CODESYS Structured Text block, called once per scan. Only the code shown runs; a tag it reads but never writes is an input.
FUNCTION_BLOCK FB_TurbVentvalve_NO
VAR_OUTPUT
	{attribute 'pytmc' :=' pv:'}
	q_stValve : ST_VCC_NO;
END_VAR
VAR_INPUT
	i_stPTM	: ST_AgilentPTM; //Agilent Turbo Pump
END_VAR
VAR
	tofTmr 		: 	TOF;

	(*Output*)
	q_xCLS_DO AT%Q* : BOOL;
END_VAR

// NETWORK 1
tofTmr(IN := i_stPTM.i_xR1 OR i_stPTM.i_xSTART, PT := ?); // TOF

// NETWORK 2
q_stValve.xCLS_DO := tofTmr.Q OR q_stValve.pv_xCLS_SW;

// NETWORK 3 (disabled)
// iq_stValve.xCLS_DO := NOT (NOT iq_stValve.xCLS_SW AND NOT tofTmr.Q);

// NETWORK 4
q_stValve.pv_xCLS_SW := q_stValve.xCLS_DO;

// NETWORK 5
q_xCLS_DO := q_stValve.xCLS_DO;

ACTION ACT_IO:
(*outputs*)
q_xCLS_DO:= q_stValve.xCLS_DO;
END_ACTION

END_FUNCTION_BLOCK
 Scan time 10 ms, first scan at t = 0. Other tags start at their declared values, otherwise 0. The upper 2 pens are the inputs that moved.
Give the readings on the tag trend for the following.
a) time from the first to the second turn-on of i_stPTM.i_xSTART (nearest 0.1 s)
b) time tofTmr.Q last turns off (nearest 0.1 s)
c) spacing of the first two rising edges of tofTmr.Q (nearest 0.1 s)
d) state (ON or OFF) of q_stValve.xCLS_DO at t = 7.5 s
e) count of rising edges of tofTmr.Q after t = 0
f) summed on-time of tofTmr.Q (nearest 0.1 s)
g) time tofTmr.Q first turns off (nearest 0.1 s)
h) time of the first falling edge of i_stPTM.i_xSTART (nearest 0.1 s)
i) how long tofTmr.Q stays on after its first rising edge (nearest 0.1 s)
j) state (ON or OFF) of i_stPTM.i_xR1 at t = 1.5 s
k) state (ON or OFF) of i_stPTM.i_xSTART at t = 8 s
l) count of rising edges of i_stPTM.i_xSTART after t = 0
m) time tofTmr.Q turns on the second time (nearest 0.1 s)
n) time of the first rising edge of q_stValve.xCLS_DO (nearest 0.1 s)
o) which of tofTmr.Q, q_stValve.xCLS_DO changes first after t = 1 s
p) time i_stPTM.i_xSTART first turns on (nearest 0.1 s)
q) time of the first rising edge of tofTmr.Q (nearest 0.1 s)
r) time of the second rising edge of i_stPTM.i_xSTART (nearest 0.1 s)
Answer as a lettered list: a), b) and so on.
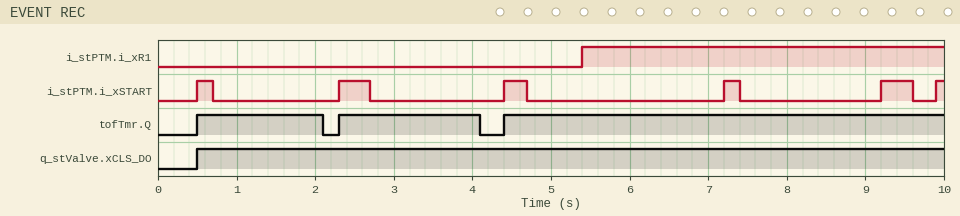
a) 1.8 s
b) 4.1 s
c) 1.8 s
d) ON
e) 3
f) 9.0 s
g) 2.1 s
h) 0.7 s
i) 1.6 s
j) OFF
k) OFF
l) 6
m) 2.3 s
n) 0.5 s
o) tofTmr.Q
p) 0.5 s
q) 0.5 s
r) 2.3 s
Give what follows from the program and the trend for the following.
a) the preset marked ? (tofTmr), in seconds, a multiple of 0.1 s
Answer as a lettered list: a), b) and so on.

a) 1.4 s
